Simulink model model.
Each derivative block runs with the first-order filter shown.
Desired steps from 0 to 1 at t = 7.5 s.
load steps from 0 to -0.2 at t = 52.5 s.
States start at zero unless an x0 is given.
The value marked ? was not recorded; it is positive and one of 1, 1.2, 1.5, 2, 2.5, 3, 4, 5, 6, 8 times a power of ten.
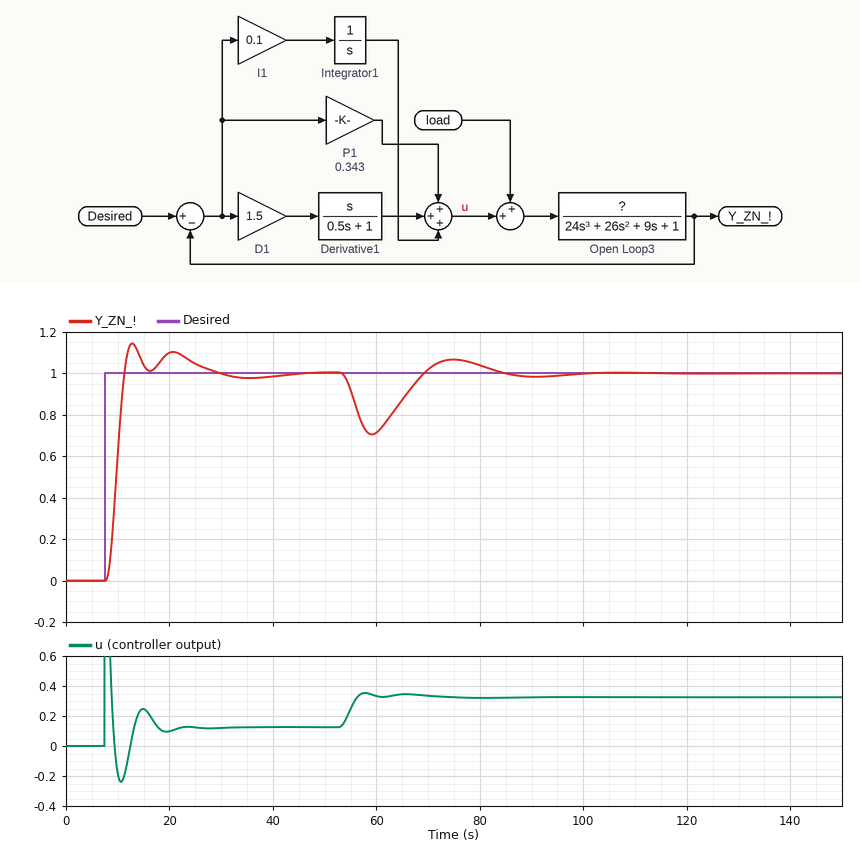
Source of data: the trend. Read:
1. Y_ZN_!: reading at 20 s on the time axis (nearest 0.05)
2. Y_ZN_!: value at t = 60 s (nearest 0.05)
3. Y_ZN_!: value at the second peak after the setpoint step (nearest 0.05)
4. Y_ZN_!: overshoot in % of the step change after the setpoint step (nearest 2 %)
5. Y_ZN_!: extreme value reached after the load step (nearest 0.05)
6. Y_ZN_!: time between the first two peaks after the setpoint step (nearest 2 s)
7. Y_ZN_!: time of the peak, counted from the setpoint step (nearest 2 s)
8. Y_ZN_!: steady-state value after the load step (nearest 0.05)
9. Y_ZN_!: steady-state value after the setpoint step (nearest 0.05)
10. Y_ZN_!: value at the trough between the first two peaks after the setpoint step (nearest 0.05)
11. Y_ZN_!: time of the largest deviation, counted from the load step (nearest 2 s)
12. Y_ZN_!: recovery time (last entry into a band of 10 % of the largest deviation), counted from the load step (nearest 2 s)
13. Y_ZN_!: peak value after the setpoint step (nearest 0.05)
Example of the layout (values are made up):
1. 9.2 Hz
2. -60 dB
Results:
1. 1.10
2. 0.70
3. 1.10
4. 14 %
5. 0.70
6. 8 s
7. 6 s
8. 1.00
9. 1.00
10. 1.00
11. 6 s
12. 28 s
13. 1.15
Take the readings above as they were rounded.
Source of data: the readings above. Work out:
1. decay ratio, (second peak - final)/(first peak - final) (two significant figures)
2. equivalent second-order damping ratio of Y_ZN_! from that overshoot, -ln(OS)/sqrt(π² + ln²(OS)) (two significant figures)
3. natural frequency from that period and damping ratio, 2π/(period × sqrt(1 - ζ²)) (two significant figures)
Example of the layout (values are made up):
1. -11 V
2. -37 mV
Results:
1. 0.67
2. 0.53
3. 0.93 rad/s
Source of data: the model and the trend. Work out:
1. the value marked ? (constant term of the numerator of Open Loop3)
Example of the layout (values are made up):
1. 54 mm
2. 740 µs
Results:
1. 8
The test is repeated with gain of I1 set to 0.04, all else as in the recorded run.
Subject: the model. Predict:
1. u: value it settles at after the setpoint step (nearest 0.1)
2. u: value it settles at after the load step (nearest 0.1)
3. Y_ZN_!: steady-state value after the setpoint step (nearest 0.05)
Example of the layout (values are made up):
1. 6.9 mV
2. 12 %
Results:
1. 0.1
2. 0.3
3. 1.00
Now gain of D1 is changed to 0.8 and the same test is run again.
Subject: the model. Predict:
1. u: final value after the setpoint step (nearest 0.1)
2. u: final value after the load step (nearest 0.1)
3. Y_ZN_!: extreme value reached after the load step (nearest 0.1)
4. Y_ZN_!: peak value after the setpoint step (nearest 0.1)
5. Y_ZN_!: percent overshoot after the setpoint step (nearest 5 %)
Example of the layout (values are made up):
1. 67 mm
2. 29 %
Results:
1. 0.1
2. 0.3
3. 0.6
4. 1.3
5. 30 %
